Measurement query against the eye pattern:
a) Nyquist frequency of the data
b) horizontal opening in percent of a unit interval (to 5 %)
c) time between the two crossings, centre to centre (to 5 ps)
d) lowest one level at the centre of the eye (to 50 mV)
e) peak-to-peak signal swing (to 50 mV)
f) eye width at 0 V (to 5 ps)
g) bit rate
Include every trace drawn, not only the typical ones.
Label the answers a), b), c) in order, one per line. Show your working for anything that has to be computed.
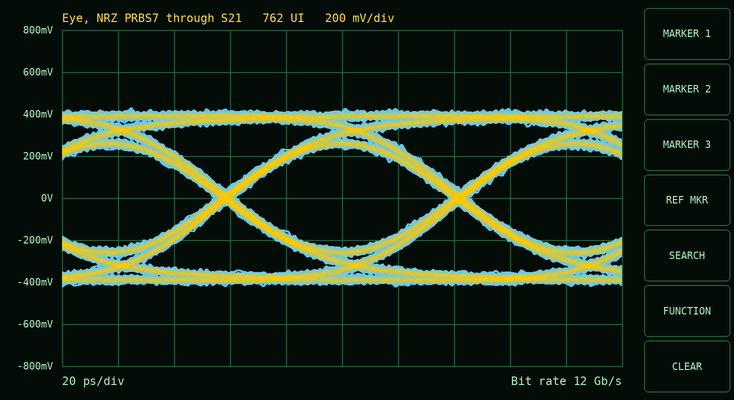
a) 6 GHz
b) 75 ps / 85 ps ≈ 88.2 %, so 90 % to the nearest 5 %
c) 85 ps
d) 250 mV
e) 850 mV
f) 75 ps
g) 12 Gb/s
